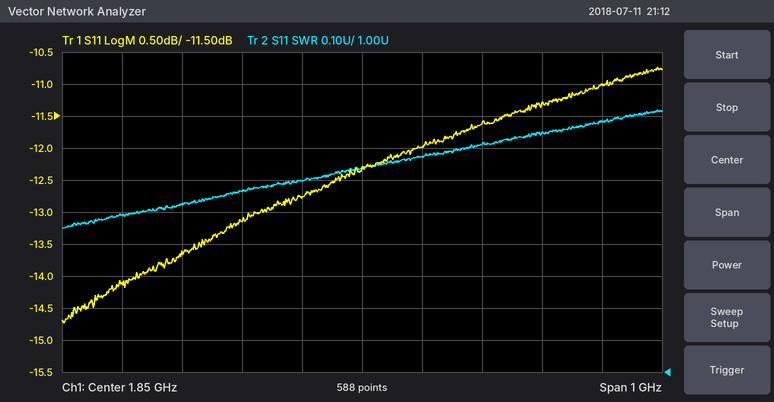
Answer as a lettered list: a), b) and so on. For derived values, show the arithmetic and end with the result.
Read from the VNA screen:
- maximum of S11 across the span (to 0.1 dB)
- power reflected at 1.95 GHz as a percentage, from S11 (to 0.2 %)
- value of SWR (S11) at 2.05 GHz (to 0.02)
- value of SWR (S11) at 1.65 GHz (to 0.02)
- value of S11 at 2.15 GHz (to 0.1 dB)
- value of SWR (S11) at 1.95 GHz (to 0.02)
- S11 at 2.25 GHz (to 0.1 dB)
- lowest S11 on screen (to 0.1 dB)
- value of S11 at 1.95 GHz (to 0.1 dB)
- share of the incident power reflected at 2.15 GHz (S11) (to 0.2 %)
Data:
a) -10.7 dB
b) 10^(-12/10) ≈ 6.31 %, so 6.4 % to the nearest 0.2 %
c) 1.72
d) 1.56
e) -11.3 dB
f) 1.68
g) -11.0 dB
h) -14.7 dB
i) -12.0 dB
j) 10^(-11.3/10) ≈ 7.4 %
